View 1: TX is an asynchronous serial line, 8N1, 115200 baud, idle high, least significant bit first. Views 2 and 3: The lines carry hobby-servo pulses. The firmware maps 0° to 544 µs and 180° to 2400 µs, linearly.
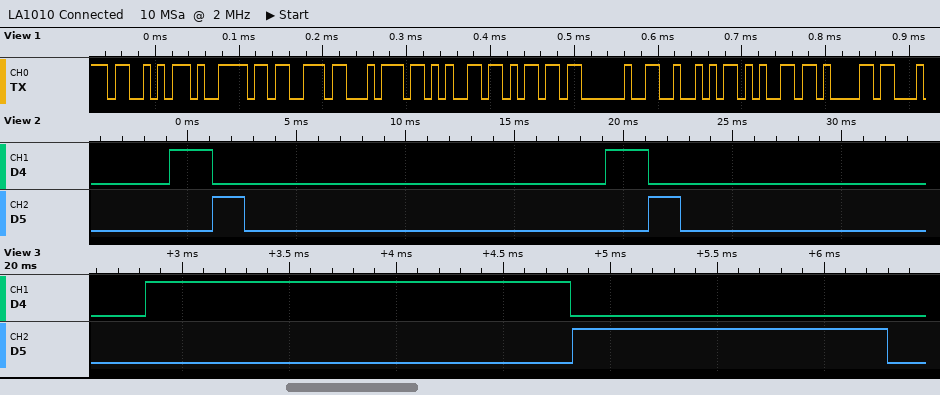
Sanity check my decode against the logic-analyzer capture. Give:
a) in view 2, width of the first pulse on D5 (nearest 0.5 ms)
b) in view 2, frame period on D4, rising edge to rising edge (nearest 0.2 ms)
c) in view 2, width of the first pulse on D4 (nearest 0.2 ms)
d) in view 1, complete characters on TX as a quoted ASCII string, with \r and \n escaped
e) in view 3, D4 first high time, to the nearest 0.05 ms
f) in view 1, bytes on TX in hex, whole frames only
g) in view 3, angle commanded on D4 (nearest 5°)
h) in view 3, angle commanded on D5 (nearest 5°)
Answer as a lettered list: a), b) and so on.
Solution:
a) 1.5 ms
b) 20.0 ms
c) 2.0 ms
d) "System Rea"
e) 2.00 ms
f) 53 79 73 74 65 6D 20 52 65 61
g) 140°
h) 90°
